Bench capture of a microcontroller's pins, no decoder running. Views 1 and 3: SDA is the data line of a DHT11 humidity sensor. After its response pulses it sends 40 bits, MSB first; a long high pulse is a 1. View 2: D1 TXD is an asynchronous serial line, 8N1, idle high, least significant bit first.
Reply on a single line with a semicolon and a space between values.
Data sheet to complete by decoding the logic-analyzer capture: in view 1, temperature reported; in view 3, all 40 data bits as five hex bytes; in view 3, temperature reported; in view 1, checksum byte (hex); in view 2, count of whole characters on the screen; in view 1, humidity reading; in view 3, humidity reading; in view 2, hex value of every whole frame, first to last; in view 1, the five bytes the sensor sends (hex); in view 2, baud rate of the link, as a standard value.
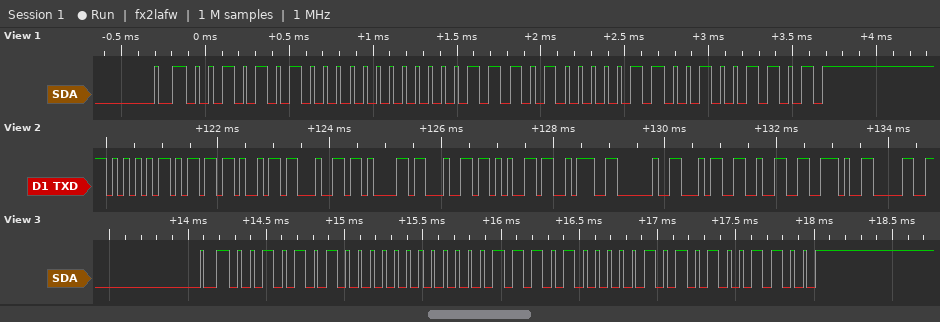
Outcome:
29.6 °C; 2A 00 1D 05 4C; 29.5 °C; 0x4D; 13; 42 %; 42 %; 55 6D 69 64 61 64 65 3A 20 34 32 2E 30; 2A 00 1D 06 4D; 9600 baud
